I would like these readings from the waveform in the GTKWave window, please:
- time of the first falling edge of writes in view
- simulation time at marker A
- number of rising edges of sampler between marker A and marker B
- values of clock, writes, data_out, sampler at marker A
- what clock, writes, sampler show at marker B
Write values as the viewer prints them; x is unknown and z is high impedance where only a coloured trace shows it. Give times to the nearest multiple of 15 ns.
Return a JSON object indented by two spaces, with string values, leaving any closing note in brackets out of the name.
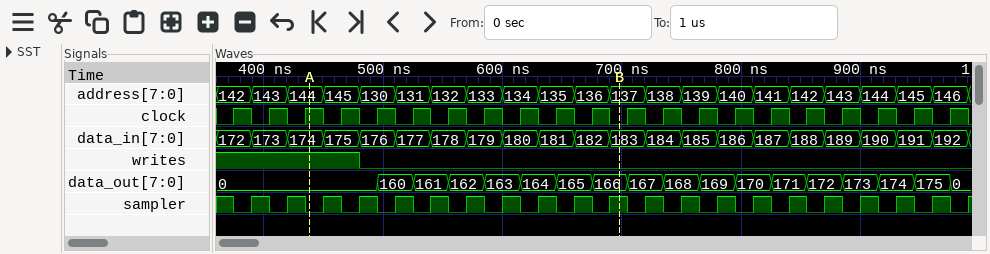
{
  "time of the first falling edge of writes in view": "480 ns",
  "simulation time at marker A": "435 ns",
  "number of rising edges of sampler between marker A and marker B": "9",
  "values of clock, writes, data_out, sampler at marker A": "clock=1, writes=1, data_out=0, sampler=0",
  "what clock, writes, sampler show at marker B": "clock=0, writes=0, sampler=1"
}
